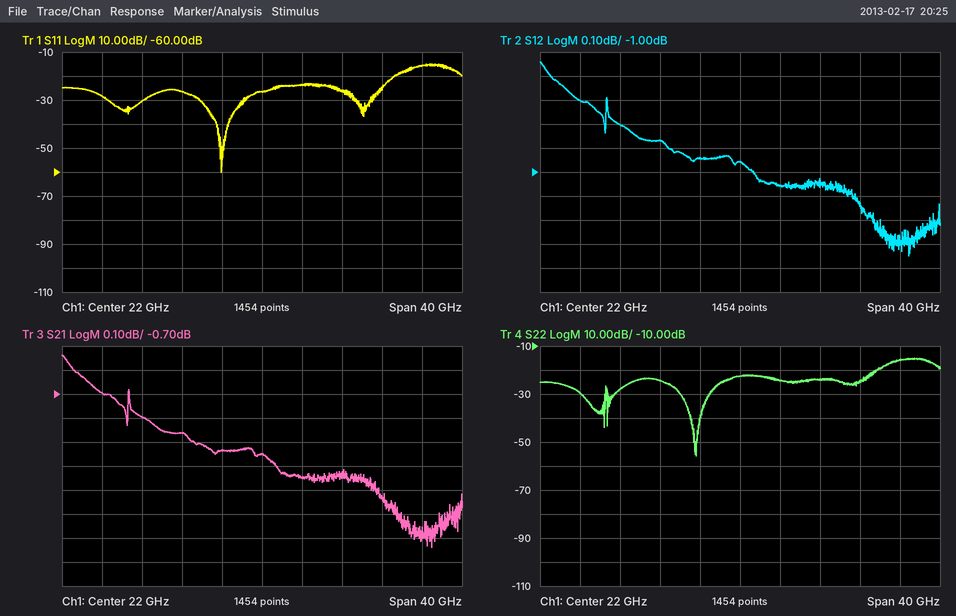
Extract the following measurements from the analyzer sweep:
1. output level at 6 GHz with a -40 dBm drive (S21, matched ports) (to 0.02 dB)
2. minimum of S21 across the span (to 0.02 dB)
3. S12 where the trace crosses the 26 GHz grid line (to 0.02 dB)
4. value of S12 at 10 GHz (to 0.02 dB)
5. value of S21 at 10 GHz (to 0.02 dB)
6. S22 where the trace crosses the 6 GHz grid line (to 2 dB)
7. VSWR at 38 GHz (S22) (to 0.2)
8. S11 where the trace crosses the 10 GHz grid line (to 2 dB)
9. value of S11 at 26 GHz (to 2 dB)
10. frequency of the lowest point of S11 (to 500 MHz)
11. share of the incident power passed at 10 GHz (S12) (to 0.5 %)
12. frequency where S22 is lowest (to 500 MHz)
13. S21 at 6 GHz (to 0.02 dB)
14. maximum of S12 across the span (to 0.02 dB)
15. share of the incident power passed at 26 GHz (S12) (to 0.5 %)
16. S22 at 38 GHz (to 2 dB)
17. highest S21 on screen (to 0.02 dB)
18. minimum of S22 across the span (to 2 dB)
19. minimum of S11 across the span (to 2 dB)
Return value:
-40.70 dBm
-1.34 dB
-1.06 dB
-0.80 dB
-0.80 dB
-30 dB
1.4
-30 dB
-24 dB
18.0 GHz
83.0 %
17.5 GHz
-0.70 dB
-0.54 dB
78.5 %
-16 dB
-0.54 dB
-56 dB
-60 dB
